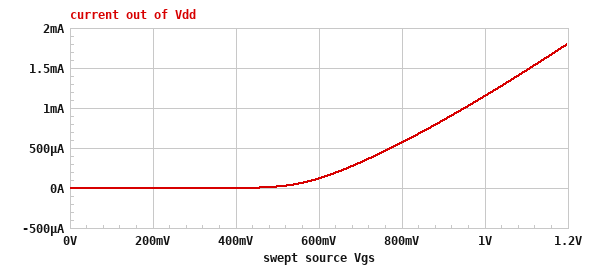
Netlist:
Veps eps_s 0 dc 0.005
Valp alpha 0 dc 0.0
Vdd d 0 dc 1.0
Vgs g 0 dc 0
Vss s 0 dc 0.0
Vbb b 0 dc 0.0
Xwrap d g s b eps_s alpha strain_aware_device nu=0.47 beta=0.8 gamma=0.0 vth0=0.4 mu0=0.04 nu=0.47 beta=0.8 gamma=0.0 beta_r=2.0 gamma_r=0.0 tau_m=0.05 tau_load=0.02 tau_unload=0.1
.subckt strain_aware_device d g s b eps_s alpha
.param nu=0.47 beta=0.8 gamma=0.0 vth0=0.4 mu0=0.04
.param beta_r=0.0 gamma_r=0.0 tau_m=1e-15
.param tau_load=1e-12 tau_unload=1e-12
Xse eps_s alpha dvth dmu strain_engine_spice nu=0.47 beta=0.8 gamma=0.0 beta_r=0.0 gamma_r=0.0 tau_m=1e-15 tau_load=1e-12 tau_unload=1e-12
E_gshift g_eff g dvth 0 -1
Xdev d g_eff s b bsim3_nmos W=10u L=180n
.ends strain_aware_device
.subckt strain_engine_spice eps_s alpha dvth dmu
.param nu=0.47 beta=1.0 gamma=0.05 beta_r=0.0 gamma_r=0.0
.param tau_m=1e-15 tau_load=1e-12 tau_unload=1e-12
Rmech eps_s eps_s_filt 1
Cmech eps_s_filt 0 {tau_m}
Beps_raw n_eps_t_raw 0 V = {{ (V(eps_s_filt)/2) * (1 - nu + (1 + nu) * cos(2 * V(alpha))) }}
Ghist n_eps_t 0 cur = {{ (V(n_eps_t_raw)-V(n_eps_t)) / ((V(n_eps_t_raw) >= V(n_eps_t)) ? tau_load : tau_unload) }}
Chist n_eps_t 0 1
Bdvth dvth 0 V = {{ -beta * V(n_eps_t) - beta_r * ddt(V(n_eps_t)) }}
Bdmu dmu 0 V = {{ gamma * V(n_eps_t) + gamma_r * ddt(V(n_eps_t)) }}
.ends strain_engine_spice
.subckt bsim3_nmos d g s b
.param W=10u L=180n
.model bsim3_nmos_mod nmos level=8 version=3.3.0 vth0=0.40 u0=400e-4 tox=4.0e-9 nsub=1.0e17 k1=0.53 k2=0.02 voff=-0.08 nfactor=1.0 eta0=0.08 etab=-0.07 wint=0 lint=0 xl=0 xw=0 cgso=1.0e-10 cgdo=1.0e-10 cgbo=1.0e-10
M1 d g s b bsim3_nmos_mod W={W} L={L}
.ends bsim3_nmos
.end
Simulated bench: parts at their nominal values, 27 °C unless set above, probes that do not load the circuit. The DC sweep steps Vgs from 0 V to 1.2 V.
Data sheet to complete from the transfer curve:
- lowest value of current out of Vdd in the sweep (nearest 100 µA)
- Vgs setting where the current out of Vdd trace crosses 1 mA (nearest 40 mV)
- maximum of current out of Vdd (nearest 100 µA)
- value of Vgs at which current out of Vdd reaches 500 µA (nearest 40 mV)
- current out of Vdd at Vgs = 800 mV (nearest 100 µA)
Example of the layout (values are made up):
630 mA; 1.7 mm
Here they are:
0 A; 960 mV; 1.8 mA; 760 mV; 600 µA
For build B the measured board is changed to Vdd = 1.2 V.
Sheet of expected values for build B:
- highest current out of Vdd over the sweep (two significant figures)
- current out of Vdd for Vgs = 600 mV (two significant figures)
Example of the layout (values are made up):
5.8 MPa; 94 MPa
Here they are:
1.9 mA; 140 µA
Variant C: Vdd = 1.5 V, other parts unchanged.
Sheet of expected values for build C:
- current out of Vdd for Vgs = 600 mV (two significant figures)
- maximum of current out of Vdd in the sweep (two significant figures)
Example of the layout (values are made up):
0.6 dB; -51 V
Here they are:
160 µA; 2.0 mA
